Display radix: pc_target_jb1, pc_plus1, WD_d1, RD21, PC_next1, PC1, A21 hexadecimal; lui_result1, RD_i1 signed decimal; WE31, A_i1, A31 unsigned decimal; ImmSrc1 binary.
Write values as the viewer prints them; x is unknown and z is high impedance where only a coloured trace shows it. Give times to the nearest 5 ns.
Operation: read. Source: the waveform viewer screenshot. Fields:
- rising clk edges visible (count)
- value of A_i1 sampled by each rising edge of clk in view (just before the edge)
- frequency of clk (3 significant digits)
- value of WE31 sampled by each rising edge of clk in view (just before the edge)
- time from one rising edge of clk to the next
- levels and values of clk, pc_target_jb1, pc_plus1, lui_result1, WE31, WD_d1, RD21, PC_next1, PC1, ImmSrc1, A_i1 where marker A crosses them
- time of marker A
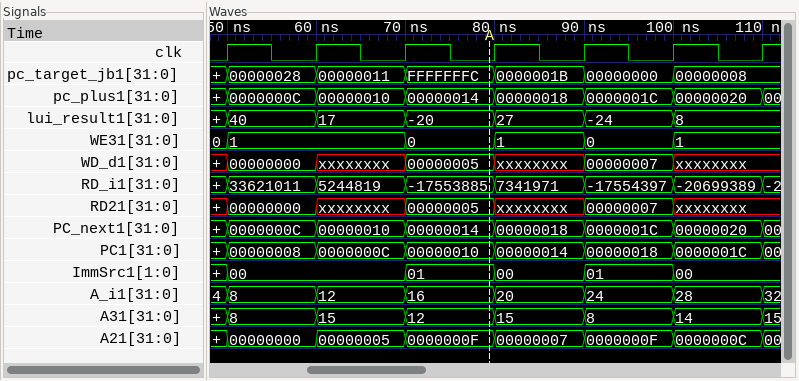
7
4, 8, 12, 16, 20, 24, 28
100 MHz
0, 1, 1, 0, 1, 0, 1
10 ns
clk=0, pc_target_jb1=FFFFFFFC, pc_plus1=00000014, lui_result1=-20, WE31=0, WD_d1=00000005, RD21=00000005, PC_next1=00000014, PC1=00000010, ImmSrc1=01, A_i1=16
80 ns
